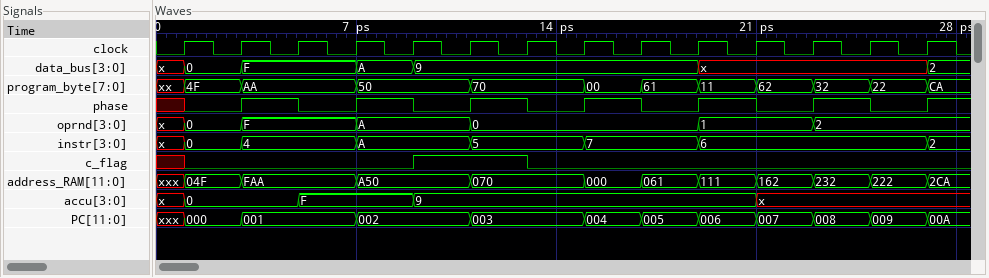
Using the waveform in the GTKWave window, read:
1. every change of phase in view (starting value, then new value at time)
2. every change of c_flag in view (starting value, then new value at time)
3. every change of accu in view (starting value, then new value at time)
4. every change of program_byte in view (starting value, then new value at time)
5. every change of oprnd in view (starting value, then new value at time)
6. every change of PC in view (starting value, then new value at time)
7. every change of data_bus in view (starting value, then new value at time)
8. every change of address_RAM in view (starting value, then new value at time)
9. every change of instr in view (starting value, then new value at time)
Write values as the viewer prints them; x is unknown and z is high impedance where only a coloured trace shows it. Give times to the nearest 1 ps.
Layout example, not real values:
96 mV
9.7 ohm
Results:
x, 0 at 1 ps, 1 at 3 ps, 0 at 5 ps, 1 at 7 ps, 0 at 9 ps, 1 at 11 ps, 0 at 13 ps, 1 at 15 ps, 0 at 17 ps, 1 at 19 ps, 0 at 21 ps, 1 at 23 ps, 0 at 25 ps, 1 at 27 ps
x, 0 at 1 ps, 1 at 9 ps, 0 at 13 ps
x, 0 at 1 ps, F at 5 ps, 9 at 9 ps, x at 21 ps
xx, 4F at 1 ps, AA at 3 ps, 50 at 7 ps, 70 at 11 ps, 00 at 15 ps, 61 at 17 ps, 11 at 19 ps, 62 at 21 ps, 32 at 23 ps, 22 at 25 ps, CA at 27 ps
x, 0 at 1 ps, F at 3 ps, A at 7 ps, 0 at 11 ps, 1 at 19 ps, 2 at 23 ps
xxx, 000 at 1 ps, 001 at 3 ps, 002 at 7 ps, 003 at 11 ps, 004 at 15 ps, 005 at 17 ps, 006 at 19 ps, 007 at 21 ps, 008 at 23 ps, 009 at 25 ps, 00A at 27 ps
x, 0 at 1 ps, F at 3 ps, A at 7 ps, 9 at 9 ps, x at 19 ps, 2 at 27 ps
xxx, 04F at 1 ps, FAA at 3 ps, A50 at 7 ps, 070 at 11 ps, 000 at 15 ps, 061 at 17 ps, 111 at 19 ps, 162 at 21 ps, 232 at 23 ps, 222 at 25 ps, 2CA at 27 ps
x, 0 at 1 ps, 4 at 3 ps, A at 7 ps, 5 at 11 ps, 7 at 15 ps, 6 at 19 ps, 2 at 27 ps
